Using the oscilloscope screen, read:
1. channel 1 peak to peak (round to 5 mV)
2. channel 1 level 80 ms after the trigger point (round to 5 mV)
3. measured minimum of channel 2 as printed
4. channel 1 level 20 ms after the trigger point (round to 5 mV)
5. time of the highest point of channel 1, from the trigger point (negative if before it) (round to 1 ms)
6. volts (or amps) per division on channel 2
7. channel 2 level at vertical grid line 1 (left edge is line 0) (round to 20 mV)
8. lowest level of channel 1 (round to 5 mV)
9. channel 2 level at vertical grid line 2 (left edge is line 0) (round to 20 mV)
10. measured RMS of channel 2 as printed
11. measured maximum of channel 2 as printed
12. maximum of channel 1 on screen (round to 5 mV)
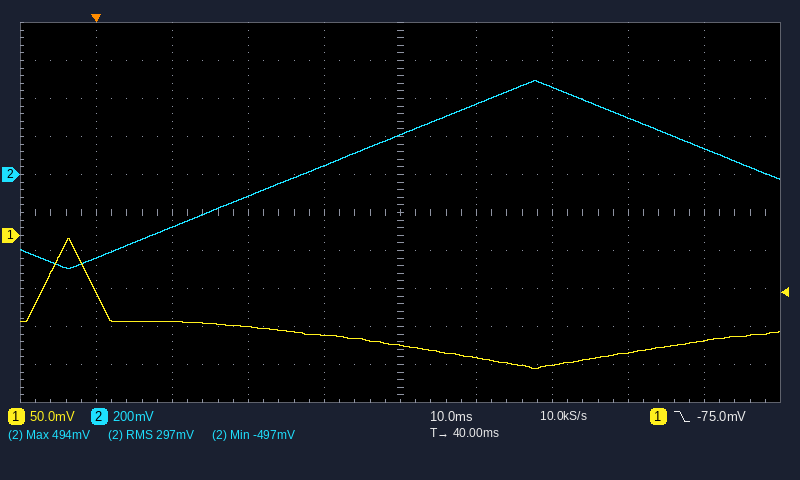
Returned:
170 mV
-140 mV
-497 mV
-120 mV
-4 ms
200 mV
-440 mV
-175 mV
-280 mV
297 mV
494 mV
-5 mV
